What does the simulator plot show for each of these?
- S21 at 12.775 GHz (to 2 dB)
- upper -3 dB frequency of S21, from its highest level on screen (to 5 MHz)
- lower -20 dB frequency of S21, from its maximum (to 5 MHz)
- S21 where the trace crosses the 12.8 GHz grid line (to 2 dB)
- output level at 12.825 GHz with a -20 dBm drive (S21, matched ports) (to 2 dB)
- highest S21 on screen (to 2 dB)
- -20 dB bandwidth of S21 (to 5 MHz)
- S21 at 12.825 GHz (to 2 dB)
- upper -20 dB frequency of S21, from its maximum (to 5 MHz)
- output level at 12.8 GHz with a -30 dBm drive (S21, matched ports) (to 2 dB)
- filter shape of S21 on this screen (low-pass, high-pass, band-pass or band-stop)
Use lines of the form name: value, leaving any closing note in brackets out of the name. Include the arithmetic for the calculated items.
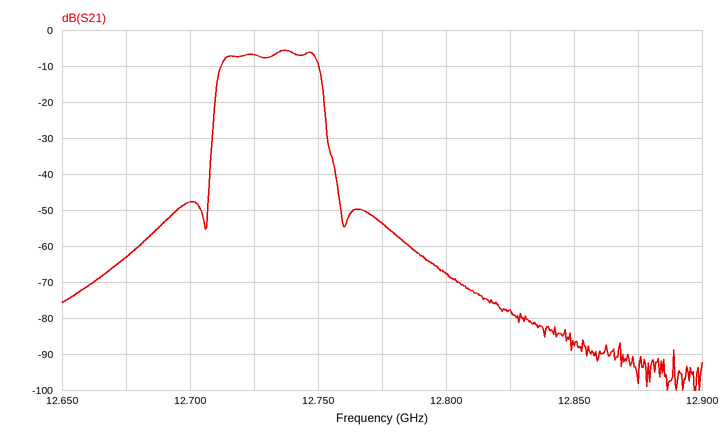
S21 at 12.775 GHz: -54 dB
upper -3 dB frequency of S21, from its highest level on screen: 12.750 GHz
lower -20 dB frequency of S21, from its maximum: 12.710 GHz
S21 where the trace crosses the 12.8 GHz grid line: -68 dB
output level at 12.825 GHz with a -20 dBm drive (S21, matched ports): -20 dBm + (-78 dB) = -98 dBm
highest S21 on screen: -6 dB
-20 dB bandwidth of S21: 12.755 GHz − 12.710 GHz = 45 MHz
S21 at 12.825 GHz: -78 dB
upper -20 dB frequency of S21, from its maximum: 12.755 GHz
output level at 12.8 GHz with a -30 dBm drive (S21, matched ports): -30 dBm + (-68 dB) = -98 dBm
filter shape of S21 on this screen: band-pass
